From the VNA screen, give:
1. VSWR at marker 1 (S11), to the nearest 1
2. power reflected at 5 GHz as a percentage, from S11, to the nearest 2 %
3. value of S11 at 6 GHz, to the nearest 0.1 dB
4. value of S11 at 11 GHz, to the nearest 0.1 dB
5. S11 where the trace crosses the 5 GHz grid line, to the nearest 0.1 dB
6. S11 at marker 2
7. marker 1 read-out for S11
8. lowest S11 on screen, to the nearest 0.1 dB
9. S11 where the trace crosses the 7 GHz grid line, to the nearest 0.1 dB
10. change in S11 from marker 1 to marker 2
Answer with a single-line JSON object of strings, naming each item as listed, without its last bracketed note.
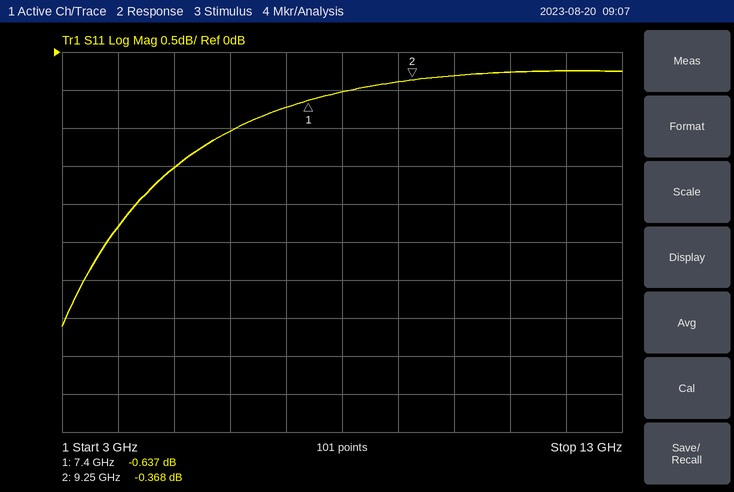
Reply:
{"VSWR at marker 1 (S11), to the nearest 1": "27", "power reflected at 5 GHz as a percentage, from S11, to the nearest 2 %": "70 %", "value of S11 at 6 GHz, to the nearest 0.1 dB": "-1.0 dB", "value of S11 at 11 GHz, to the nearest 0.1 dB": "-0.3 dB", "S11 where the trace crosses the 5 GHz grid line, to the nearest 0.1 dB": "-1.5 dB", "S11 at marker 2": "-0.368 dB", "marker 1 read-out for S11": "-0.637 dB", "lowest S11 on screen, to the nearest 0.1 dB": "-3.6 dB", "S11 where the trace crosses the 7 GHz grid line, to the nearest 0.1 dB": "-0.7 dB", "change in S11 from marker 1 to marker 2": "0.269 dB"}
